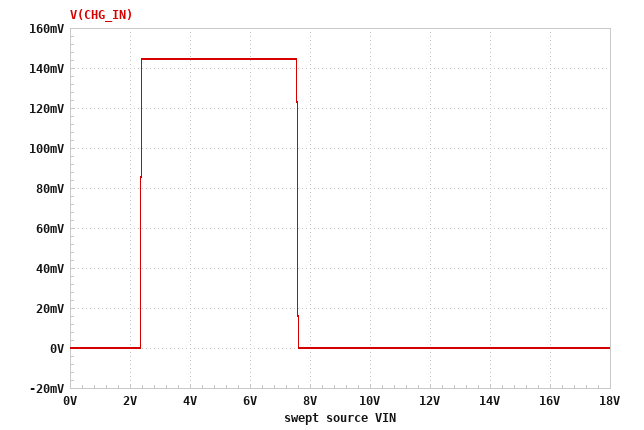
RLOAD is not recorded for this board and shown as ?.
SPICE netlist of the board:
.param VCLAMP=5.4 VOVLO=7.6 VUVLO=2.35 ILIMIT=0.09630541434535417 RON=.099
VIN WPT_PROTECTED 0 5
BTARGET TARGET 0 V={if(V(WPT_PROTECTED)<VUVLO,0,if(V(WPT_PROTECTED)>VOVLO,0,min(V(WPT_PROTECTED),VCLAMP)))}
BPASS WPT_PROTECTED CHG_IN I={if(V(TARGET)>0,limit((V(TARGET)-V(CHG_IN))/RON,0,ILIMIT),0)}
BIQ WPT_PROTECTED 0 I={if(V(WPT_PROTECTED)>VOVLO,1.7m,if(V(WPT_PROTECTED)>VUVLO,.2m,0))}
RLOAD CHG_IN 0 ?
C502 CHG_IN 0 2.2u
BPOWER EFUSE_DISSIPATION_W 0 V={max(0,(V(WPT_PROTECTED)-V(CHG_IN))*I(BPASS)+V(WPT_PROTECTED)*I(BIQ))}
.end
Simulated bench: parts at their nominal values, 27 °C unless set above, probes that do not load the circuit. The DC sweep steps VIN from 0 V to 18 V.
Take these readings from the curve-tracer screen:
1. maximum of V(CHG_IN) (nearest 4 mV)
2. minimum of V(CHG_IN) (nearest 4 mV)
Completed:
144 mV
0 V
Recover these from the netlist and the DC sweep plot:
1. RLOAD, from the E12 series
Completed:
1.5 Ω
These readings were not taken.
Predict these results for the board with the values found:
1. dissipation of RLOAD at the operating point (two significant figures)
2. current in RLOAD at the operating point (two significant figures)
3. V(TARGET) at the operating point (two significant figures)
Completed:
14 mW
96 mA
5.0 V
